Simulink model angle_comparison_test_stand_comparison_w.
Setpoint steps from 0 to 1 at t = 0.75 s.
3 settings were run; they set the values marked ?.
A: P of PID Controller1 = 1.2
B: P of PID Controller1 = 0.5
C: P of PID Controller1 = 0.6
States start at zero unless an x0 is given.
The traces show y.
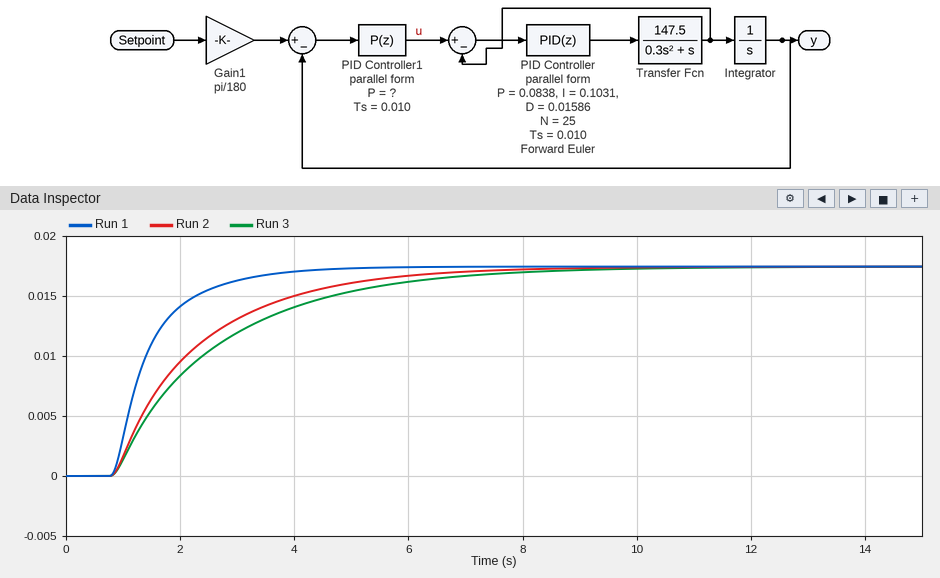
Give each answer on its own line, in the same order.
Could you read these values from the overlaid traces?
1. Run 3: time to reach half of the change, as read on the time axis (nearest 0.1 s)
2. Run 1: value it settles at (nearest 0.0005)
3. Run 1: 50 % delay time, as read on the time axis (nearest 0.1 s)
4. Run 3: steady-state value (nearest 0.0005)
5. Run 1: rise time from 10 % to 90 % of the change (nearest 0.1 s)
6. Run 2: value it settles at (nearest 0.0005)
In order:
2.1 s
0.0175
1.3 s
0.0175
1.7 s
0.0175
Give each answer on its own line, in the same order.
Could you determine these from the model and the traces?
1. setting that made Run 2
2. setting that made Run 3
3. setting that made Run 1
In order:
C
B
A
